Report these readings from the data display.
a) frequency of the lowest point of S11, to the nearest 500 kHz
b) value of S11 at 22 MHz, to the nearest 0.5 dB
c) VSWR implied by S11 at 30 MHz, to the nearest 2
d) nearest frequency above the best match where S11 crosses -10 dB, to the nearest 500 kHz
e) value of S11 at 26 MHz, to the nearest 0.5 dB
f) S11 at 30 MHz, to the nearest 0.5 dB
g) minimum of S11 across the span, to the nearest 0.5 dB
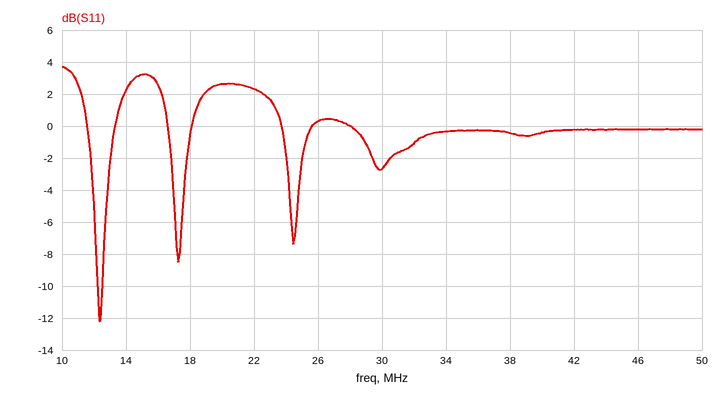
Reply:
12.5 MHz
2.5 dB
6
12.5 MHz
0.5 dB
-2.5 dB
-12.0 dB
